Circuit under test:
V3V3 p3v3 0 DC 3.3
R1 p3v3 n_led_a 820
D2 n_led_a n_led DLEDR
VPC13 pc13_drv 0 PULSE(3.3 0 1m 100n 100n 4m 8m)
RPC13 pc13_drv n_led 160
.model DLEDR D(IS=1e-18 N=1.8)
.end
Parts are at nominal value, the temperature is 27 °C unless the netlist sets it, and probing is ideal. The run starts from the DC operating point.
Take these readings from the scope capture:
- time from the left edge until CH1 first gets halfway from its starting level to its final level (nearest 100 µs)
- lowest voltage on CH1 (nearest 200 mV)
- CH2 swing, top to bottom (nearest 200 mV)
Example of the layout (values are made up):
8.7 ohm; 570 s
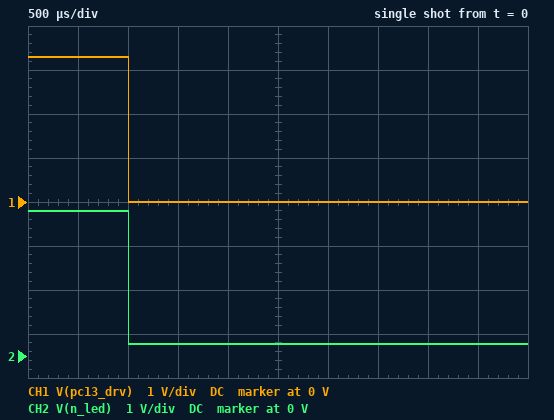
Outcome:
1.0 ms; 0 V; 3.0 V
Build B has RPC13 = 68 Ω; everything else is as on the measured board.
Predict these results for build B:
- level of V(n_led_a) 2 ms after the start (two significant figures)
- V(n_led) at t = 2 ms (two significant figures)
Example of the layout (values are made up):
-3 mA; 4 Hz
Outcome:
1.8 V; 130 mV
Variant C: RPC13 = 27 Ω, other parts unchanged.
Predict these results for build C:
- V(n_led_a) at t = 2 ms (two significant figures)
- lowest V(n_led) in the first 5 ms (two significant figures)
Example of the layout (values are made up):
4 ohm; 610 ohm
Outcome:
1.7 V; 53 mV
